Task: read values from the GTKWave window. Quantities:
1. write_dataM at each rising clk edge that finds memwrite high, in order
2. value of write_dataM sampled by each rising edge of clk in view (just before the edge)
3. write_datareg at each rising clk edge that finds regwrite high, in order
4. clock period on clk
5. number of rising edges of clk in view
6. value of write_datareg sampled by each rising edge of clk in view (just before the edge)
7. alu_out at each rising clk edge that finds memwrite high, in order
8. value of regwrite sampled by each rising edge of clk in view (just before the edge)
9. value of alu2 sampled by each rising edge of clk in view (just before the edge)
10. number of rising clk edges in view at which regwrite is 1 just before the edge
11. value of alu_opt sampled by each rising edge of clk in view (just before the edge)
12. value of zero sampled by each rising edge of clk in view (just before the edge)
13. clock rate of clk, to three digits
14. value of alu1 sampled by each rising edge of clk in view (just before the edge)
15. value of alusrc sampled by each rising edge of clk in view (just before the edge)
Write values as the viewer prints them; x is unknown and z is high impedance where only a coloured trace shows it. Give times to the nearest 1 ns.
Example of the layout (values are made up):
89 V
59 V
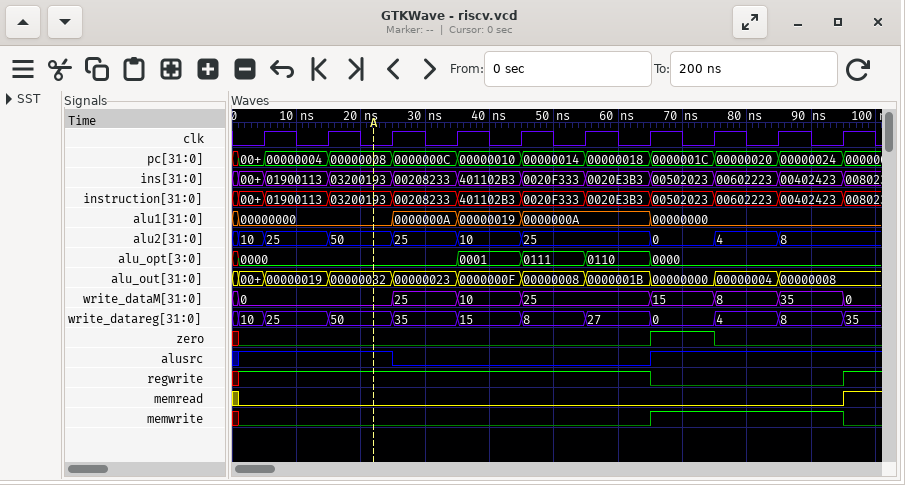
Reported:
15, 8, 35
0, 0, 0, 25, 10, 25, 25, 15, 8, 35
10, 25, 50, 35, 15, 8, 27
10 ns
10
10, 25, 50, 35, 15, 8, 27, 0, 4, 8
00000000, 00000004, 00000008
1 1 1 1 1 1 1 0 0 0
10, 25, 50, 25, 10, 25, 25, 0, 4, 8
7
0000, 0000, 0000, 0000, 0001, 0111, 0110, 0000, 0000, 0000
0 0 0 0 0 0 0 1 0 0
100 MHz
00000000, 00000000, 00000000, 0000000A, 00000019, 0000000A, 0000000A, 00000000, 00000000, 00000000
1 1 1 0 0 0 0 1 1 1
